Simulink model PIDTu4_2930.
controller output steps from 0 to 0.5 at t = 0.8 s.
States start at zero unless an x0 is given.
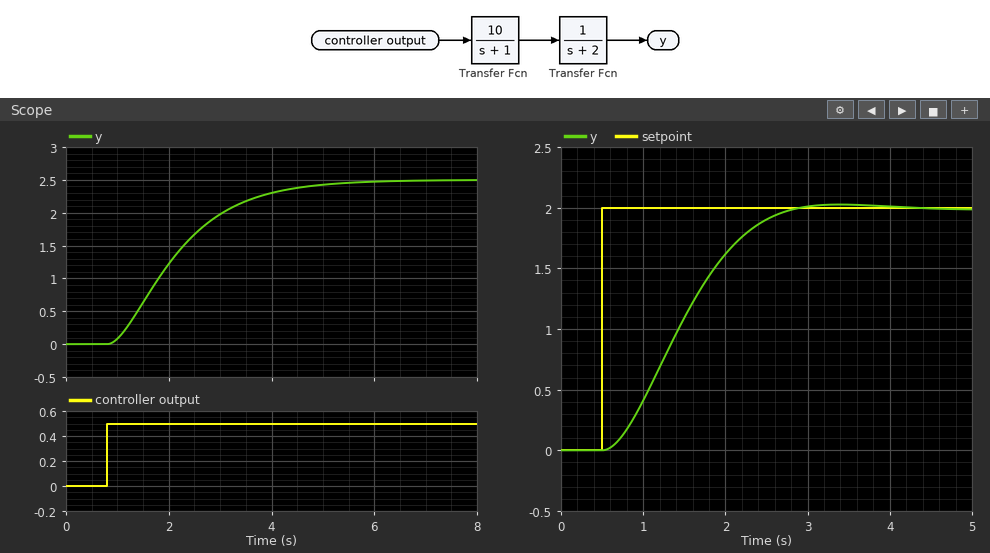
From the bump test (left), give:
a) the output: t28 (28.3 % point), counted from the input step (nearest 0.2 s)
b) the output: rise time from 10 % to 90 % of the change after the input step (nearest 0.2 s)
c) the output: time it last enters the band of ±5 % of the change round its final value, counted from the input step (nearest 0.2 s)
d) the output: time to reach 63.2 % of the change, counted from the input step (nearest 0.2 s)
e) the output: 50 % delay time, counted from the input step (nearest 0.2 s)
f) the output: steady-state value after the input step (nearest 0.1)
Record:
0.8 s
2.6 s
3.6 s
1.6 s
1.2 s
2.5
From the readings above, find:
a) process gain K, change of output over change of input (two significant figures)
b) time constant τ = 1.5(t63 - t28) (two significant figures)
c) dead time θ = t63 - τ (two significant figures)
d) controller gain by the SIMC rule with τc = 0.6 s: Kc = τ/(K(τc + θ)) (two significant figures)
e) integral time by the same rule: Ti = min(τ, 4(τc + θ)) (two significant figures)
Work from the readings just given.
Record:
5.0
1.2 s
0.40 s
0.24
1.2 s
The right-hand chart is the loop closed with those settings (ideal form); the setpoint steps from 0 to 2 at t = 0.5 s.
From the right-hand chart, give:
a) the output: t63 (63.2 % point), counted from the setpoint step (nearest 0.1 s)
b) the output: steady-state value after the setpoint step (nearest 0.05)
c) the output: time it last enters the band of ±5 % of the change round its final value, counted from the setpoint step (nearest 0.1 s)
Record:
1.1 s
2.00
2.0 s
